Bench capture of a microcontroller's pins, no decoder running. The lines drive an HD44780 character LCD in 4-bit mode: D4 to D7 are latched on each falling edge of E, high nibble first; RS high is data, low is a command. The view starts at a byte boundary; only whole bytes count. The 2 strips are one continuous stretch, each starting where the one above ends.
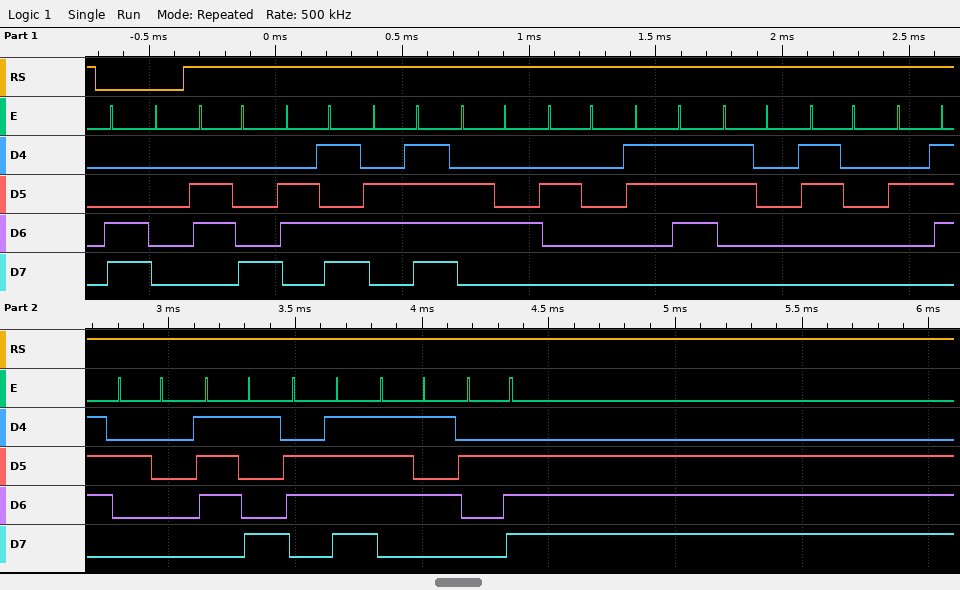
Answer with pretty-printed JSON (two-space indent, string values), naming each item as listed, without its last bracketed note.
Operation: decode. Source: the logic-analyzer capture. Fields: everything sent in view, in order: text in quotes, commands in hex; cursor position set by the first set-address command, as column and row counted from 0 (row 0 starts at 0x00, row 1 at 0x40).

{
  "everything sent in view, in order: text in quotes, commands in hex": "0xC0 \"hmod 700' you.\"",
  "cursor position set by the first set-address command, as column and row counted from 0": "column 0, row 1"
}
